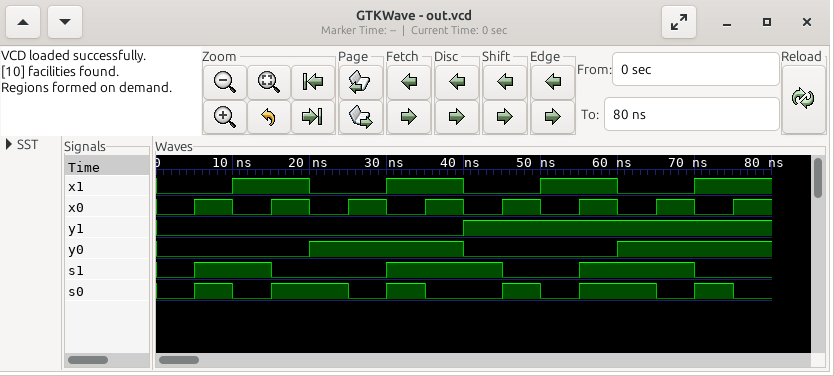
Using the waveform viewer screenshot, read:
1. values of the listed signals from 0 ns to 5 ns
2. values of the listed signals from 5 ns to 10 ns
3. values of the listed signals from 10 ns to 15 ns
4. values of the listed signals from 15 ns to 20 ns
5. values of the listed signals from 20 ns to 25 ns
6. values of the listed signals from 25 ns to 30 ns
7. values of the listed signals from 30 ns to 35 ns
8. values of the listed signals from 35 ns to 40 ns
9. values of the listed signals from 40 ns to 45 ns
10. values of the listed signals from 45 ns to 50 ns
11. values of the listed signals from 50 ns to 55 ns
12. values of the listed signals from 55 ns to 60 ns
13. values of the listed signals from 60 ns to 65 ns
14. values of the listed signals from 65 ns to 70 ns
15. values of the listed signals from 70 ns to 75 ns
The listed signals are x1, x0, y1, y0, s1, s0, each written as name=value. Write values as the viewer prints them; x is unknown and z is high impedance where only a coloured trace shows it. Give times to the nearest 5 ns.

x1=0, x0=0, y1=0, y0=0, s1=0, s0=0
x1=0, x0=1, y1=0, y0=0, s1=1, s0=1
x1=1, x0=0, y1=0, y0=0, s1=1, s0=0
x1=1, x0=1, y1=0, y0=0, s1=0, s0=1
x1=0, x0=0, y1=0, y0=1, s1=0, s0=1
x1=0, x0=1, y1=0, y0=1, s1=0, s0=0
x1=1, x0=0, y1=0, y0=1, s1=1, s0=1
x1=1, x0=1, y1=0, y0=1, s1=1, s0=0
x1=0, x0=0, y1=1, y0=0, s1=1, s0=0
x1=0, x0=1, y1=1, y0=0, s1=0, s0=1
x1=1, x0=0, y1=1, y0=0, s1=0, s0=0
x1=1, x0=1, y1=1, y0=0, s1=1, s0=1
x1=0, x0=0, y1=1, y0=1, s1=1, s0=1
x1=0, x0=1, y1=1, y0=1, s1=1, s0=0
x1=1, x0=0, y1=1, y0=1, s1=0, s0=1
